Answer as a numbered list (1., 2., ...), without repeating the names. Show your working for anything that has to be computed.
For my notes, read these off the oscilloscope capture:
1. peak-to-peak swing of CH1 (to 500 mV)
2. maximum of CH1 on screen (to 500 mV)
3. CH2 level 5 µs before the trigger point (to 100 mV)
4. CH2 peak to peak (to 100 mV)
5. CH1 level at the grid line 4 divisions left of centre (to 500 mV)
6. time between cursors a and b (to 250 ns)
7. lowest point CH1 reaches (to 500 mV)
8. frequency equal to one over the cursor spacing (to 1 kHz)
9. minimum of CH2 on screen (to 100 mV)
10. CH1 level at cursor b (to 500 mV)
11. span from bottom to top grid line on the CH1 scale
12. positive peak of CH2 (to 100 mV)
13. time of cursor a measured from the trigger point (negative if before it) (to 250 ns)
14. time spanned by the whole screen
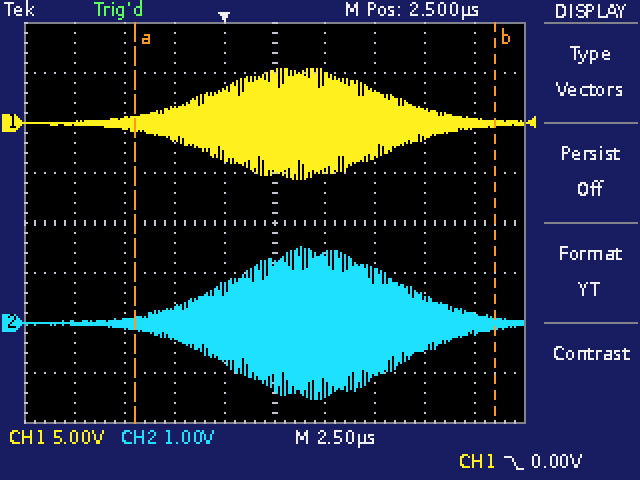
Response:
1. 5.5 V − (-5.5 V) = 11.0 V
2. 5.5 V
3. 0.0 V
4. 1.5 V − (-1.5 V) = 3.0 V
5. 0.0 V
6. 18.00 µs
7. -5.5 V
8. 1 / 18.00 µs ≈ 56 kHz
9. -1.5 V
10. 0.0 V
11. 40 V
12. 1.5 V
13. -4.50 µs
14. 25 µs
